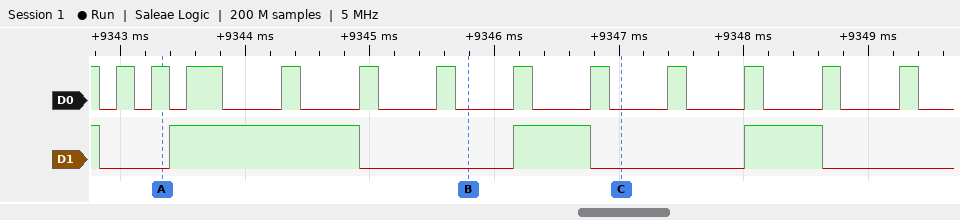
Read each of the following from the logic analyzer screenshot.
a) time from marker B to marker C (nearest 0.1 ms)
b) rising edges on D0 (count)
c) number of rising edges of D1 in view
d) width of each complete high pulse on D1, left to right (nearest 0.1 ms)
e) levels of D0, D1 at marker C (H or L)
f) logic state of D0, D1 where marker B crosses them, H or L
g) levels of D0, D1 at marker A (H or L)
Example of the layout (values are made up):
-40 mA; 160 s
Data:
1.2 ms; 12; 3; 1.5 ms, 0.6 ms, 0.6 ms; D0=L, D1=L; D0=L, D1=L; D0=H, D1=L
